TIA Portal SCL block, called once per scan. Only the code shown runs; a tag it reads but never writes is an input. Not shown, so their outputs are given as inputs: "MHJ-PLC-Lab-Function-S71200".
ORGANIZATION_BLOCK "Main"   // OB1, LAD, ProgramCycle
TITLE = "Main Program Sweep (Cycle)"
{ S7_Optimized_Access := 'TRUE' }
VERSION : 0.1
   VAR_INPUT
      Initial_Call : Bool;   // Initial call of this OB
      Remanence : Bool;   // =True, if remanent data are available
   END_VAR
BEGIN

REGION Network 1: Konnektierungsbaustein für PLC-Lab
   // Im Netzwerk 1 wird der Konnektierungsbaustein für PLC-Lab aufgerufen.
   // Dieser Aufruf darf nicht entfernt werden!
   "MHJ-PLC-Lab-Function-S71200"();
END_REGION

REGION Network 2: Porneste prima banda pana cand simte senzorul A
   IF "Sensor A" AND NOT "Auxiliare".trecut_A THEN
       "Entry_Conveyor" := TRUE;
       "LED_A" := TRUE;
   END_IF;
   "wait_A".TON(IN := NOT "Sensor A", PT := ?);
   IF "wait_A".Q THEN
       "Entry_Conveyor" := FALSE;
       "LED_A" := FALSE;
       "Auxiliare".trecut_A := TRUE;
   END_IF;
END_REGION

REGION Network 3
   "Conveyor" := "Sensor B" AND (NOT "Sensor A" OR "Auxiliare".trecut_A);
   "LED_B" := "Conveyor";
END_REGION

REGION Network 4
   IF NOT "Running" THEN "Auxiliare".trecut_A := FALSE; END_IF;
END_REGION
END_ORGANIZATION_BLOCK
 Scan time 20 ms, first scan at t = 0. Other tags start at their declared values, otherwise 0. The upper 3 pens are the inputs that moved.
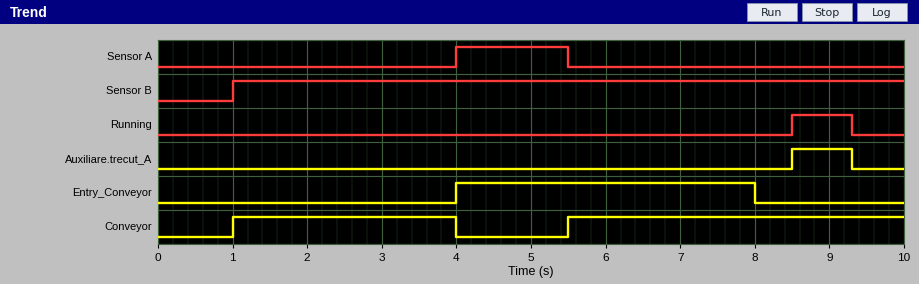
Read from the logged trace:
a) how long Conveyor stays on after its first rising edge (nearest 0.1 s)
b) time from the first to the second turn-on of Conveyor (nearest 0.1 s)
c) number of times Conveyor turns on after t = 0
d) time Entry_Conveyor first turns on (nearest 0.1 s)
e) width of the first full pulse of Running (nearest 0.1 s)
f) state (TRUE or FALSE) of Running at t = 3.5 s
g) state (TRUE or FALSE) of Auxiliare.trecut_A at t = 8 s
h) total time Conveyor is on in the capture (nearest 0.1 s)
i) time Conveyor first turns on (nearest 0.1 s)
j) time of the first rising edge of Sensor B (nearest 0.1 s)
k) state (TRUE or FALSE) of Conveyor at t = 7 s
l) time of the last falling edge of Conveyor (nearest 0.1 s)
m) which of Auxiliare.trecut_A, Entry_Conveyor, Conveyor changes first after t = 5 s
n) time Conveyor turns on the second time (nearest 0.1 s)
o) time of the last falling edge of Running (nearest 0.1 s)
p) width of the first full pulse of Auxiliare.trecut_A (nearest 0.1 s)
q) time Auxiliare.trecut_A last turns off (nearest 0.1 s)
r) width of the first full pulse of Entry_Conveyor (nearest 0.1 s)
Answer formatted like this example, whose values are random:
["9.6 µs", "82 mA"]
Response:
["3.0 s", "4.5 s", "2", "4.0 s", "0.8 s", "FALSE", "FALSE", "7.5 s", "1.0 s", "1.0 s", "TRUE", "4.0 s", "Conveyor", "5.5 s", "9.3 s", "0.8 s", "9.3 s", "4.0 s"]
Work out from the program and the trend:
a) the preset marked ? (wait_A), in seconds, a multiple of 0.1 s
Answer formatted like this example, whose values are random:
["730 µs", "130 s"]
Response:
["2.5 s"]
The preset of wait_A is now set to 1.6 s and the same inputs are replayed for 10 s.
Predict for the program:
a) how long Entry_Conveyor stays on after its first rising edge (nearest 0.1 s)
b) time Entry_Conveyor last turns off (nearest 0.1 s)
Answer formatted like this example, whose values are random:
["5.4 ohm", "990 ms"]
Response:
["3.1 s", "7.1 s"]
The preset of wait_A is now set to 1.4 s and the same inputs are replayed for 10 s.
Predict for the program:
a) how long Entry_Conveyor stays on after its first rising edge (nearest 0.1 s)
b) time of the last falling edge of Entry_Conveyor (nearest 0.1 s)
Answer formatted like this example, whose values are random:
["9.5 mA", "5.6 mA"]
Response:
["2.9 s", "6.9 s"]
